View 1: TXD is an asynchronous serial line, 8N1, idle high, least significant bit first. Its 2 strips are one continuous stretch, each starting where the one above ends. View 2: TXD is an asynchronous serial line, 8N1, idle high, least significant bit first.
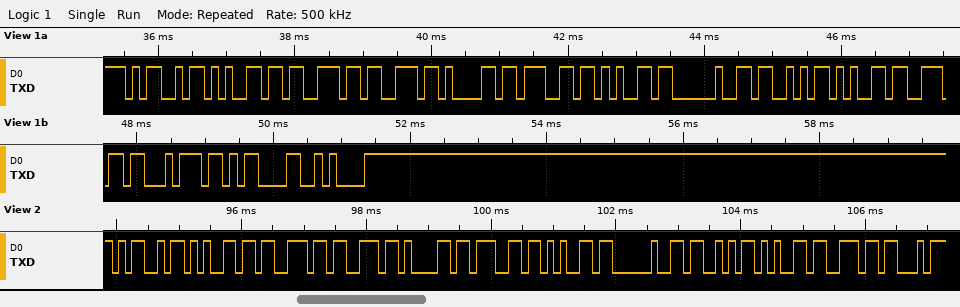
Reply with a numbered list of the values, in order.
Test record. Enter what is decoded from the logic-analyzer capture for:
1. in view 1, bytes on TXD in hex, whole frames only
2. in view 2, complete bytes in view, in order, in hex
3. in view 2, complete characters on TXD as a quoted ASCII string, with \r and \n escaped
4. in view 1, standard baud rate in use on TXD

1. 4D 65 73 73 61 67 65 20 53 65 6E 74 0D 0A
2. 0x4D 0x65 0x73 0x73 0x61 0x67 0x65 0x20 0x53 0x65 0x6E
3. "Message Sen"
4. 9600 baud
